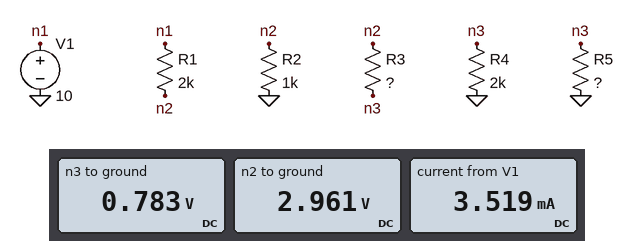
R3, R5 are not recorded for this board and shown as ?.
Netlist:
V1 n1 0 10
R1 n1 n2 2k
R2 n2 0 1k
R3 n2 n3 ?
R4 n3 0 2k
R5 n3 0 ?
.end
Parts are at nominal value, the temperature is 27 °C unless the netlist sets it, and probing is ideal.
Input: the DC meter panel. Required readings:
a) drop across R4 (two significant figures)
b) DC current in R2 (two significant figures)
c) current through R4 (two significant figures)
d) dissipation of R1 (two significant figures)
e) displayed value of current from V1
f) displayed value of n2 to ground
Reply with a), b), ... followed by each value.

a) 780 mV
b) 3.0 mA
c) 390 µA
d) 25 mW
e) 3.519 mA
f) 2.961 V
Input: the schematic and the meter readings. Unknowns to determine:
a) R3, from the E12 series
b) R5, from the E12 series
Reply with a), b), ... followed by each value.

a) 3.9 kΩ
b) 4.7 kΩ
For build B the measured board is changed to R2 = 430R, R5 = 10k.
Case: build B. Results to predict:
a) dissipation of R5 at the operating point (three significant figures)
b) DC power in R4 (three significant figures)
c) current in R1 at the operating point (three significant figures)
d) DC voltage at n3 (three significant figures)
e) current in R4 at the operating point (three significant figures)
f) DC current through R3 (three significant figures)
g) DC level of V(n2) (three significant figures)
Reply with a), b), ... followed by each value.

a) 24.8 µW
b) 124 µW
c) 4.17 mA
d) 498 mV
e) 249 µA
f) 299 µA
g) 1.66 V
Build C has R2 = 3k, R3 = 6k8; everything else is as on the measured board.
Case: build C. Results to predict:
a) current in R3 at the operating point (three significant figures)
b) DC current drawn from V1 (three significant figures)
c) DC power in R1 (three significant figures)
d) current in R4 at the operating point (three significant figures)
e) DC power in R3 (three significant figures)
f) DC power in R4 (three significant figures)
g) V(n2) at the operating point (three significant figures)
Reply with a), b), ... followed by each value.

a) 638 µA
b) 2.38 mA
c) 11.4 mW
d) 448 µA
e) 2.77 mW
f) 401 µW
g) 5.23 V
